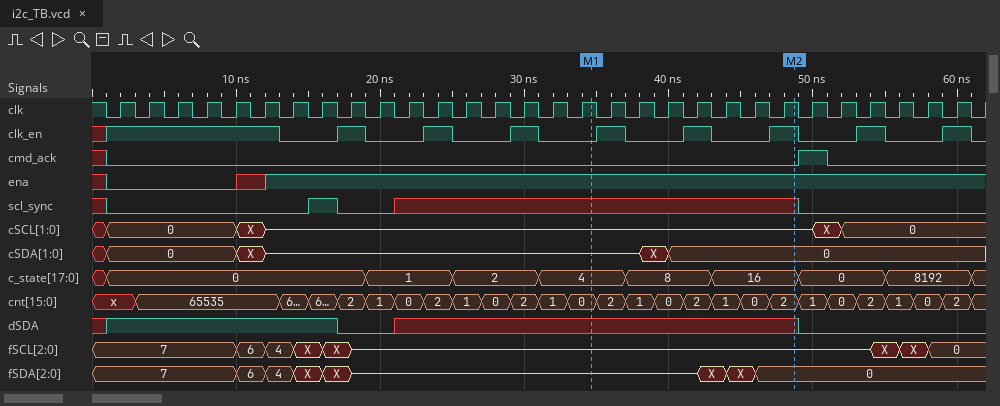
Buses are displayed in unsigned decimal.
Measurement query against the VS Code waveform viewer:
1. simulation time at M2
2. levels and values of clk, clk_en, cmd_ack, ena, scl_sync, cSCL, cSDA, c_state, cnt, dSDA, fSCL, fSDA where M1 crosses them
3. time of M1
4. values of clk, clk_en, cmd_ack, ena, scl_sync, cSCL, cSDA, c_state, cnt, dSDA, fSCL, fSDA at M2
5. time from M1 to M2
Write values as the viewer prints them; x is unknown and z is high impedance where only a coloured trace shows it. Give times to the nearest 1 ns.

49 ns
clk=1, clk_en=0, cmd_ack=0, ena=1, scl_sync=x, cSCL=z, cSDA=z, c_state=4, cnt=0, dSDA=x, fSCL=z, fSDA=z
35 ns
clk=1, clk_en=1, cmd_ack=0, ena=1, scl_sync=x, cSCL=z, cSDA=0, c_state=16, cnt=2, dSDA=x, fSCL=z, fSDA=0
14 ns
